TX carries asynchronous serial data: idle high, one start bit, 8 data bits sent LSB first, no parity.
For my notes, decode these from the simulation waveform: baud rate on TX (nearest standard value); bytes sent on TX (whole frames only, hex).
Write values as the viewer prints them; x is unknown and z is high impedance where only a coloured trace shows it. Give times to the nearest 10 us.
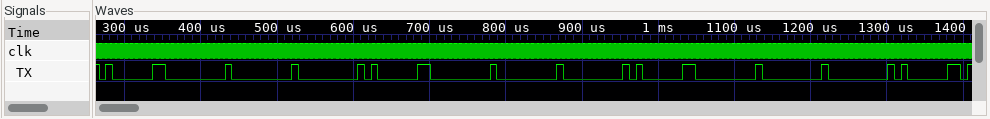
115200 baud
81, 00, 00, 00, 81, 00, 00, 00, 81, 00, 00, 00, 81
